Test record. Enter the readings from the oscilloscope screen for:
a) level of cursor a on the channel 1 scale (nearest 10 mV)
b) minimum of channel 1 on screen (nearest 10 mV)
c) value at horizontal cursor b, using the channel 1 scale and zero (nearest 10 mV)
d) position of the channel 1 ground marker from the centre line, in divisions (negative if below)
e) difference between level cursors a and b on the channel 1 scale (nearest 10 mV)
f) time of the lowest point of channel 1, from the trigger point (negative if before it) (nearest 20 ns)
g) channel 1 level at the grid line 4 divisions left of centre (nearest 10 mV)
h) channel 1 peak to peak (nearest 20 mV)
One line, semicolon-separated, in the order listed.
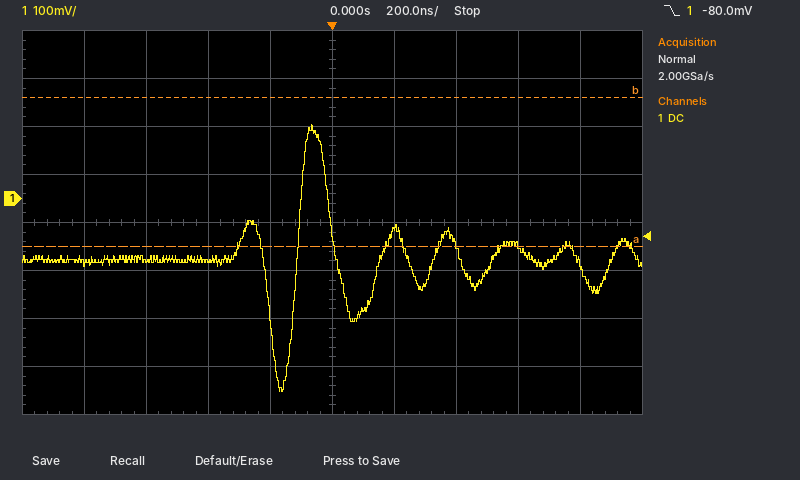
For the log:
-100 mV; -400 mV; 210 mV; +0.5 div; 310 mV; -160 ns; -130 mV; 560 mV
